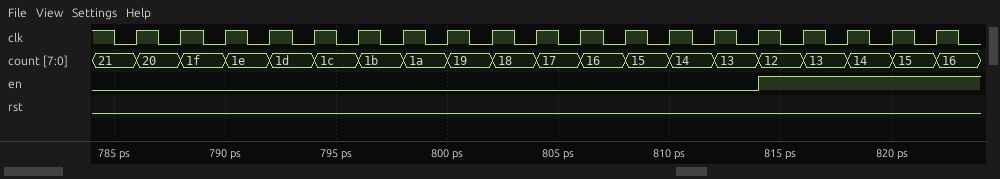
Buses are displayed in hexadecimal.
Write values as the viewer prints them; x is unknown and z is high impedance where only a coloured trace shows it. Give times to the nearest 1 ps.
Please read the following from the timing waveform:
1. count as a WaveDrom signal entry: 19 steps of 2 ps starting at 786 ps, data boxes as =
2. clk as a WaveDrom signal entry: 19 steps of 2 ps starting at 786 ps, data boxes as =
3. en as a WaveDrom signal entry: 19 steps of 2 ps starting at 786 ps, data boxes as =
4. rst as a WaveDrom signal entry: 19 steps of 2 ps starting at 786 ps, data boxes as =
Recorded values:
{name: 'count', wave: '===================', data: '20 1f 1e 1d 1c 1b 1a 19 18 17 16 15 14 13 12 13 14 15 16'}
{name: 'clk', wave: 'p..................'}
{name: 'en', wave: '0.............1....'}
{name: 'rst', wave: '0..................'}
